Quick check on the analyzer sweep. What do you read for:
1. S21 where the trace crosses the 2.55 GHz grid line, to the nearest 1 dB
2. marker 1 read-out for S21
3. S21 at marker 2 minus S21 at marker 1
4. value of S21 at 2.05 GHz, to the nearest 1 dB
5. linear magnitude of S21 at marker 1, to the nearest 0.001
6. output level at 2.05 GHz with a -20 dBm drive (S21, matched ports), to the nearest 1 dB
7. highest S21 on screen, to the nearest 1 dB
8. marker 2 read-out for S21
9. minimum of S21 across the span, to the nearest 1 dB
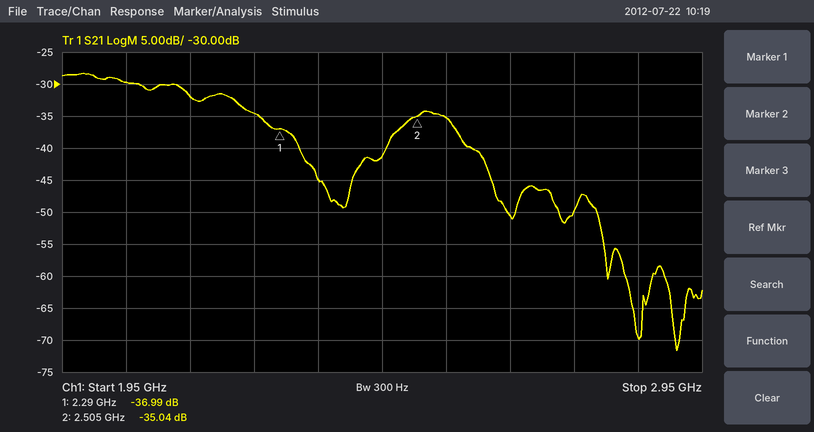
-35 dB
-36.99 dB
1.95 dB
-30 dB
0.014
-50 dBm
-28 dB
-35.04 dB
-72 dB
